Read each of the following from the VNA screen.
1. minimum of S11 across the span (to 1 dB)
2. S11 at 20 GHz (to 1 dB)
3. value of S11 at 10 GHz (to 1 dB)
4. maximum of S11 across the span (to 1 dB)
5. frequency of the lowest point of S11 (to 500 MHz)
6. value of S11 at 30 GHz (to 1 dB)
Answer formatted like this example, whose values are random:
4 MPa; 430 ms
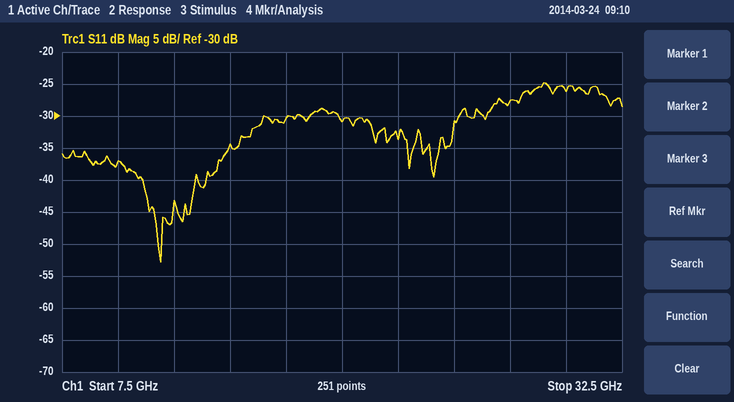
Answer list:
-53 dB; -31 dB; -37 dB; -25 dB; 12.0 GHz; -26 dB
